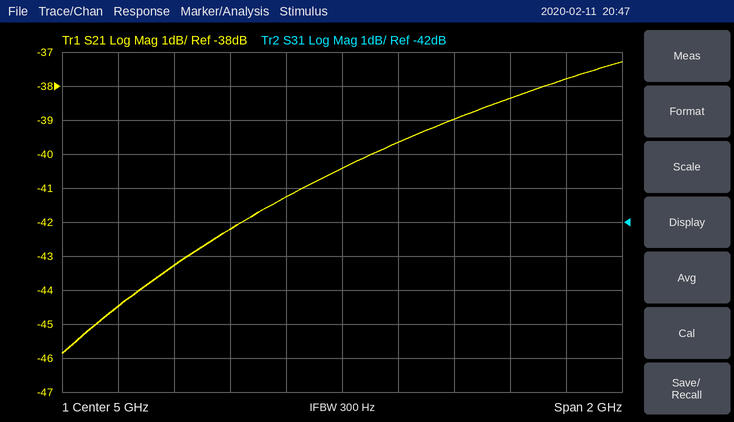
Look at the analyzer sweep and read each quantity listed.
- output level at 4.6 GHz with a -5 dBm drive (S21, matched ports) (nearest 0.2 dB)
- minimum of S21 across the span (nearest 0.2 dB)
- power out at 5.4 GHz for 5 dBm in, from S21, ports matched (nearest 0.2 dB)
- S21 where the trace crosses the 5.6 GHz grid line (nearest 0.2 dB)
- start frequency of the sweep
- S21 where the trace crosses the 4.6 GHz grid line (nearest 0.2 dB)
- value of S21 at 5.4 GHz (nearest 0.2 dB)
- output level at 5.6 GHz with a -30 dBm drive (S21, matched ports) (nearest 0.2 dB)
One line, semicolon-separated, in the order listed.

-47.2 dBm; -45.8 dB; -34.0 dBm; -38.4 dB; 4 GHz; -42.2 dB; -39.0 dB; -68.4 dBm
